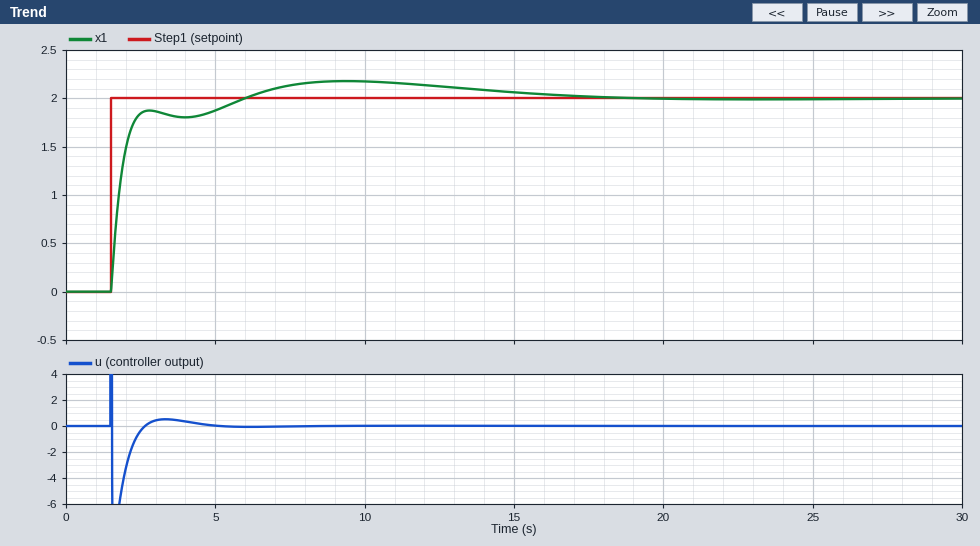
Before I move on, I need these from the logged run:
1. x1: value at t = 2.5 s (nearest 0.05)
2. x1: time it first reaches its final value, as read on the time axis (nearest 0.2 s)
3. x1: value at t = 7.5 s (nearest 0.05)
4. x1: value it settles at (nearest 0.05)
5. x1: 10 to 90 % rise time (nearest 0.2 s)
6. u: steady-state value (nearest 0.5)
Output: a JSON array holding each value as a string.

["1.85", "6.0 s", "2.15", "2.00", "0.8 s", "0.0"]
